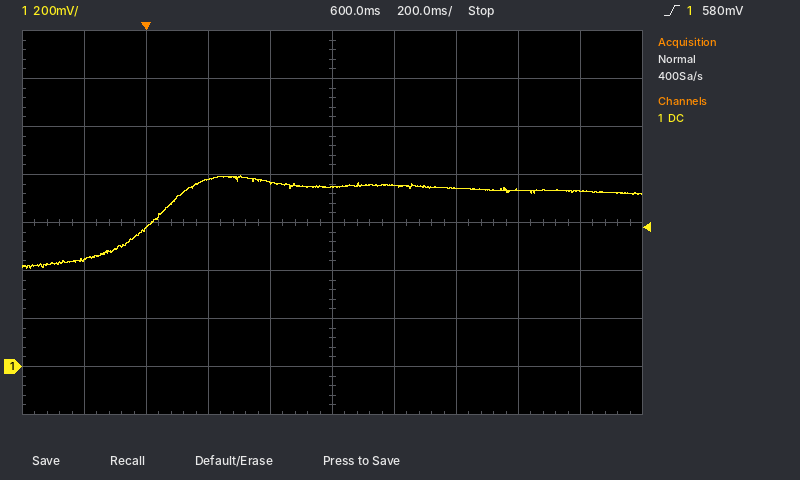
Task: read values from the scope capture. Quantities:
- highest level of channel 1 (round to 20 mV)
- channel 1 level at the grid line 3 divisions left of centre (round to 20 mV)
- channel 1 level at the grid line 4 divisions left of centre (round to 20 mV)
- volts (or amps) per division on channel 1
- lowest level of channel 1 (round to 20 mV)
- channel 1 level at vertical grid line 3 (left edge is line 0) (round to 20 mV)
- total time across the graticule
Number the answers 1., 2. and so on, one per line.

1. 800 mV
2. 580 mV
3. 440 mV
4. 200 mV
5. 400 mV
6. 780 mV
7. 2 s
